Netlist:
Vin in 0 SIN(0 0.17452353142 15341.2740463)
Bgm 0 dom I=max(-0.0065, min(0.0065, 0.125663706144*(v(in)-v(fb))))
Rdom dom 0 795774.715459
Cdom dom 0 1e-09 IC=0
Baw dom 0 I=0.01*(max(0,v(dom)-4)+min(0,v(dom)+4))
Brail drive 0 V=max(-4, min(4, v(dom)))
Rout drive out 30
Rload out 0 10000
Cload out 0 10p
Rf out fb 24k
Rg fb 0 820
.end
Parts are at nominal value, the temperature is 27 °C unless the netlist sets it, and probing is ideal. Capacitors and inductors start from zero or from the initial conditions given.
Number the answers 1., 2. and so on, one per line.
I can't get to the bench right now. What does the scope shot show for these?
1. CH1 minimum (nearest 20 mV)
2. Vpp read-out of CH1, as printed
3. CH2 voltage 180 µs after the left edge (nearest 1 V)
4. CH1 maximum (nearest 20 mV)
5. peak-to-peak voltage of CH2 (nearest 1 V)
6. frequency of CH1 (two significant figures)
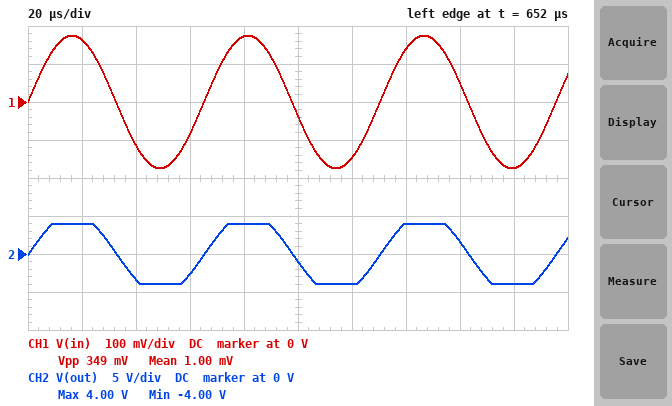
1. -180 mV
2. 349 mV
3. -4 V
4. 180 mV
5. 8 V
6. 15 kHz
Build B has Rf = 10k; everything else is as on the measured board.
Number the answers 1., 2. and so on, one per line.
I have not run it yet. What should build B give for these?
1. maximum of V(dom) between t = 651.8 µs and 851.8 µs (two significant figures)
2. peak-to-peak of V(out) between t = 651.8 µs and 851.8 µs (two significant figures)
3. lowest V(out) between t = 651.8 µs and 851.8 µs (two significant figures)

1. 2.3 V
2. 4.6 V
3. -2.3 V
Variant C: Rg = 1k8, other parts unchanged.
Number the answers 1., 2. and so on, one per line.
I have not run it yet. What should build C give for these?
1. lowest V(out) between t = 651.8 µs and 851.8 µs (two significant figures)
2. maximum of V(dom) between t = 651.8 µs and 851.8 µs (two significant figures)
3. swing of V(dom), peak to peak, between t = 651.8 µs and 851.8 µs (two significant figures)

1. -2.5 V
2. 2.5 V
3. 5.0 V
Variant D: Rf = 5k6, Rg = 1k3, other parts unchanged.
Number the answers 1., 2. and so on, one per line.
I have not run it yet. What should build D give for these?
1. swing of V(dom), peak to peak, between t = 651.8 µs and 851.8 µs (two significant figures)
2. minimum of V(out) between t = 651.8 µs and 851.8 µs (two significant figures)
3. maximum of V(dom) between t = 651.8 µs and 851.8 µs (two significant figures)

1. 1.9 V
2. -930 mV
3. 930 mV
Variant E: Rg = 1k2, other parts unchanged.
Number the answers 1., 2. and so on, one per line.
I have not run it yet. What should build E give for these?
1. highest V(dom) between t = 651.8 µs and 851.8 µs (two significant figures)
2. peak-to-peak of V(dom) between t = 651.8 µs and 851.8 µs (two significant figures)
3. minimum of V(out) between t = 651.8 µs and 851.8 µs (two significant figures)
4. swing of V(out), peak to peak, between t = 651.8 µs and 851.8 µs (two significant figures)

1. 3.7 V
2. 7.4 V
3. -3.7 V
4. 7.3 V
